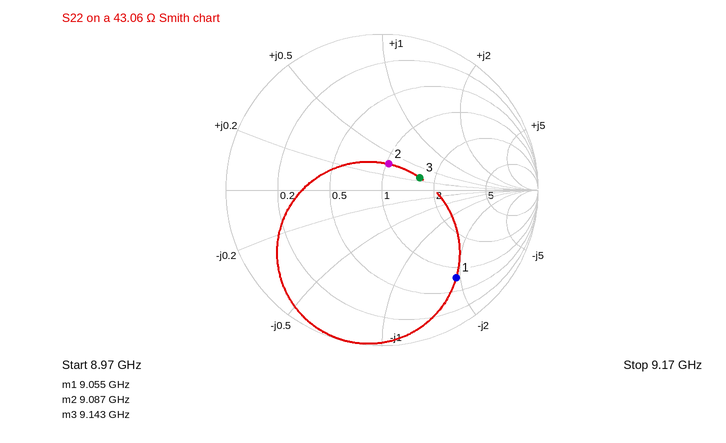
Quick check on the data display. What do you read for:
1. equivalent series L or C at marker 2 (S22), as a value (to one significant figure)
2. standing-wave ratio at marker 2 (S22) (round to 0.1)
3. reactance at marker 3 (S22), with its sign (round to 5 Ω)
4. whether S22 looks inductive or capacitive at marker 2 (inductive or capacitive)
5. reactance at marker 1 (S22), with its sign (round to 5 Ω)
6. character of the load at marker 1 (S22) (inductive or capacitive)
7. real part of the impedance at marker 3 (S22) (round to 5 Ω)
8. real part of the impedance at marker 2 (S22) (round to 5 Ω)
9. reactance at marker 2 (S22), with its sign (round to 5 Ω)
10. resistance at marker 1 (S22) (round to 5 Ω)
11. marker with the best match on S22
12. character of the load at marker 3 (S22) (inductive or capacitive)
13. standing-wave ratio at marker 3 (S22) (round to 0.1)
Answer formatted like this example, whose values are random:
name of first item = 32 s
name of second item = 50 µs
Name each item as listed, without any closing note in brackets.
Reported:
equivalent series L or C at marker 2 (S22), as a value = 300 pH
standing-wave ratio at marker 2 (S22) = 1.4
reactance at marker 3 (S22), with its sign = +10 Ω
whether S22 looks inductive or capacitive at marker 2 = inductive
reactance at marker 1 (S22), with its sign = -80 Ω
character of the load at marker 1 (S22) = capacitive
real part of the impedance at marker 3 (S22) = 70 Ω
real part of the impedance at marker 2 (S22) = 45 Ω
reactance at marker 2 (S22), with its sign = +15 Ω
resistance at marker 1 (S22) = 35 Ω
marker with the best match on S22 = marker 2
character of the load at marker 3 (S22) = inductive
standing-wave ratio at marker 3 (S22) = 1.7
